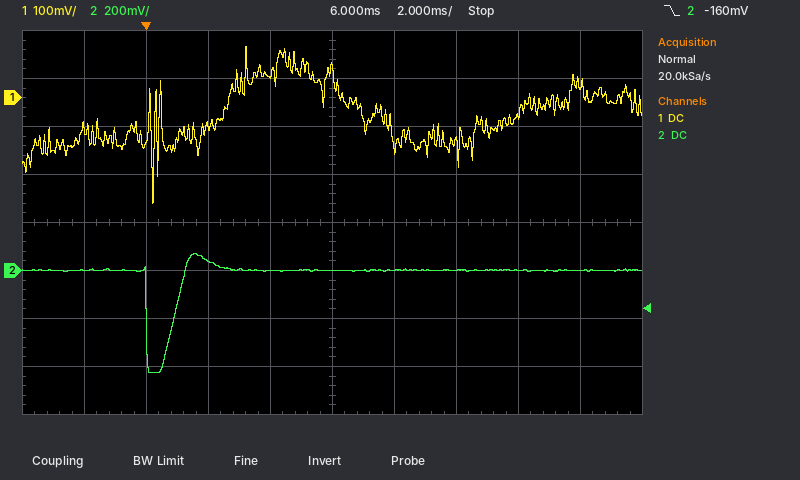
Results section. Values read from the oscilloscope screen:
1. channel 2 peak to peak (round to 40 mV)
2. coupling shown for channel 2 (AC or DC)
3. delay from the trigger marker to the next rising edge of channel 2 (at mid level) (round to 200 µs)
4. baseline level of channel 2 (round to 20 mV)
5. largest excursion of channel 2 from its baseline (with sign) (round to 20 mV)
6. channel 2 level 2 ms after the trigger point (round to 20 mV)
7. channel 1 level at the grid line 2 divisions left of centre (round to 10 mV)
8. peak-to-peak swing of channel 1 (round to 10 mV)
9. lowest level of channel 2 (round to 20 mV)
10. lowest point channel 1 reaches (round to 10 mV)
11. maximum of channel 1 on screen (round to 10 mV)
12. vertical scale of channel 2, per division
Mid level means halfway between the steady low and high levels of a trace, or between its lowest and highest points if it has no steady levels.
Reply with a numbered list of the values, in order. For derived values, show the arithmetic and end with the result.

1. 480 mV
2. DC
3. 1.0 ms
4. 0 mV
5. -420 mV − (0 mV) = -420 mV
6. 40 mV
7. -60 mV
8. 110 mV − (-220 mV) = 330 mV
9. -420 mV
10. -220 mV
11. 110 mV
12. 200 mV
